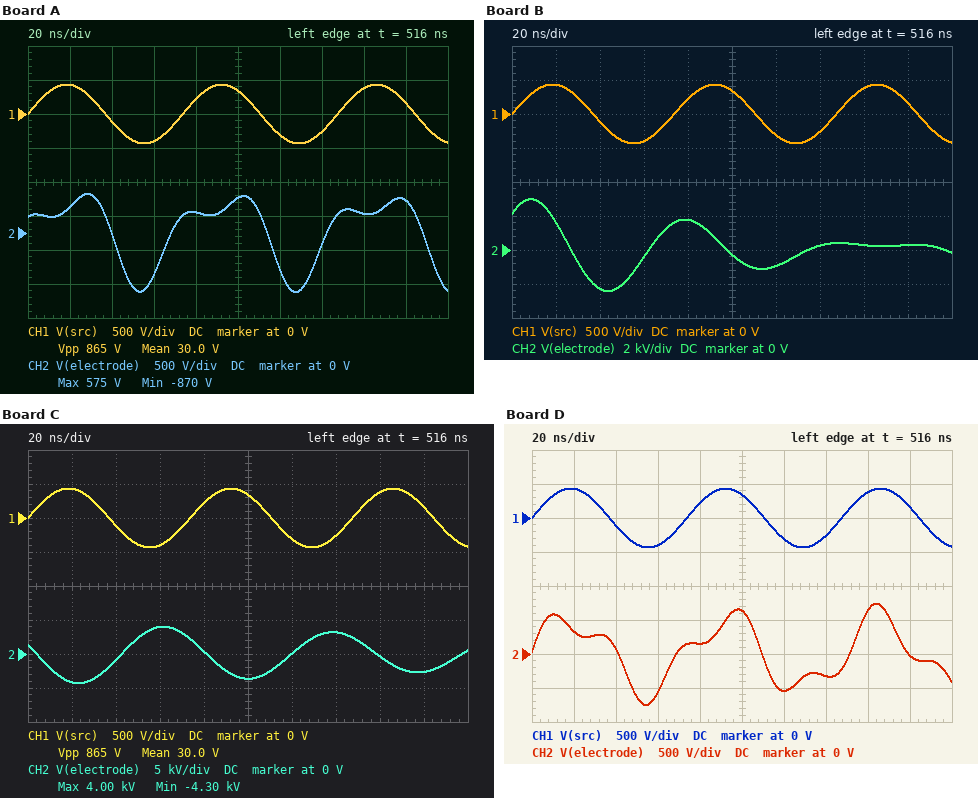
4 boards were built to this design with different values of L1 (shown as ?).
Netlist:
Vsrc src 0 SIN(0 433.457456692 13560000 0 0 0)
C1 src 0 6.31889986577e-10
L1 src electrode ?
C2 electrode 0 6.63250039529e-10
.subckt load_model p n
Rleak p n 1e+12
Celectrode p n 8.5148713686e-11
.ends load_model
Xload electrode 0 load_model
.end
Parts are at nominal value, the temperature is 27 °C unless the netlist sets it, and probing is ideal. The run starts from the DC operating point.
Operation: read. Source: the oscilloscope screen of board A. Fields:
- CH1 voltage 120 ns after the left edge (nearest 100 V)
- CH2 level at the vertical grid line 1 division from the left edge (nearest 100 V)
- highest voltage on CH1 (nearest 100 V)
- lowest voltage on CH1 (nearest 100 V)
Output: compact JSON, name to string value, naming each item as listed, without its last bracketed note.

{"CH1 voltage 120 ns after the left edge": "-300 V", "CH2 level at the vertical grid line 1 division from the left edge": "400 V", "highest voltage on CH1": "400 V", "lowest voltage on CH1": "-400 V"}
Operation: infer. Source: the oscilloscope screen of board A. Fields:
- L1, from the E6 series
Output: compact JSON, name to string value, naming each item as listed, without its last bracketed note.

{"L1, from the E6 series": "47 nH"}
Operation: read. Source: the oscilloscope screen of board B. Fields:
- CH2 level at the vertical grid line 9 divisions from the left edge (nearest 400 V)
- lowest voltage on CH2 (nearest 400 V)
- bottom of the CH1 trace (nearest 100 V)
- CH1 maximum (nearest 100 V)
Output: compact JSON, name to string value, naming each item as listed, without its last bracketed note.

{"CH2 level at the vertical grid line 9 divisions from the left edge": "400 V", "lowest voltage on CH2": "-2.4 kV", "bottom of the CH1 trace": "-400 V", "CH1 maximum": "400 V"}
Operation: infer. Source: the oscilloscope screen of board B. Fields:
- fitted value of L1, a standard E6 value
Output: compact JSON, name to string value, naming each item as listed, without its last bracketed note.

{"fitted value of L1, a standard E6 value": "150 nH"}
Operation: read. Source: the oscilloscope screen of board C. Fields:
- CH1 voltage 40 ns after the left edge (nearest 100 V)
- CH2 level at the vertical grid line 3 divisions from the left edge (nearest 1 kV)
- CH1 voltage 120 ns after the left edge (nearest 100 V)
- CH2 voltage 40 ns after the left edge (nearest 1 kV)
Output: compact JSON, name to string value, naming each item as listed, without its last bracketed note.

{"CH1 voltage 40 ns after the left edge": "-100 V", "CH2 level at the vertical grid line 3 divisions from the left edge": "4 kV", "CH1 voltage 120 ns after the left edge": "-300 V", "CH2 voltage 40 ns after the left edge": "-1 kV"}
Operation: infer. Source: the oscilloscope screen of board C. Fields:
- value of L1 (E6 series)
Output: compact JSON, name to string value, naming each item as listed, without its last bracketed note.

{"value of L1": "220 nH"}
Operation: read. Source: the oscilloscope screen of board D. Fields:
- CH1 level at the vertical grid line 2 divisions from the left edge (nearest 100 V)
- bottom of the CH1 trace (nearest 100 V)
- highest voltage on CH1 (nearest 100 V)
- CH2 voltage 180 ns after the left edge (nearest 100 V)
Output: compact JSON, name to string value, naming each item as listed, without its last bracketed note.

{"CH1 level at the vertical grid line 2 divisions from the left edge": "-100 V", "bottom of the CH1 trace": "-400 V", "highest voltage on CH1": "400 V", "CH2 voltage 180 ns after the left edge": "0 V"}
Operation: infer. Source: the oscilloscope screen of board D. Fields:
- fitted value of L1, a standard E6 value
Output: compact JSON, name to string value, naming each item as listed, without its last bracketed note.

{"fitted value of L1, a standard E6 value": "33 nH"}
